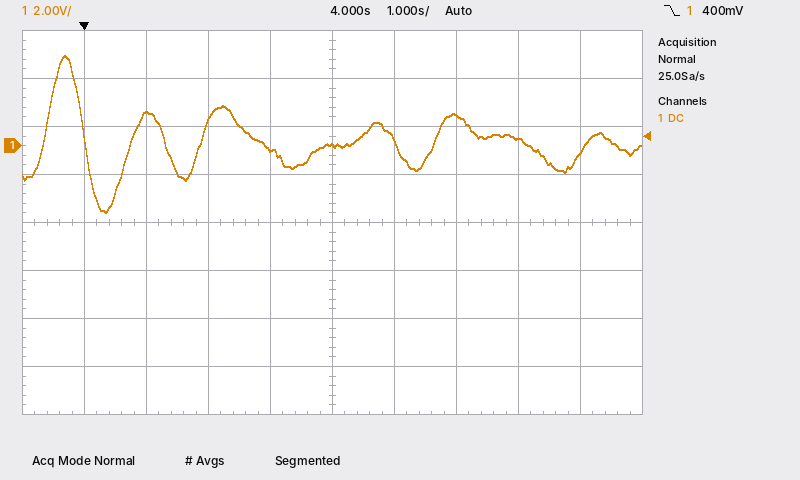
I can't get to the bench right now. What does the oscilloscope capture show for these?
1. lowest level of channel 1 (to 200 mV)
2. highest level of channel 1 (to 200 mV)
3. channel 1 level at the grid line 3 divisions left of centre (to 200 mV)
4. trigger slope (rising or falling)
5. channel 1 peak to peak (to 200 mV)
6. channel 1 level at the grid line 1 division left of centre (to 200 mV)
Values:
-2.8 V
3.8 V
1.4 V
falling
6.6 V
-200 mV
